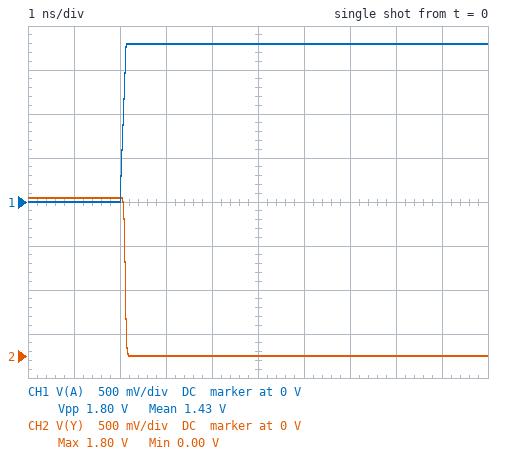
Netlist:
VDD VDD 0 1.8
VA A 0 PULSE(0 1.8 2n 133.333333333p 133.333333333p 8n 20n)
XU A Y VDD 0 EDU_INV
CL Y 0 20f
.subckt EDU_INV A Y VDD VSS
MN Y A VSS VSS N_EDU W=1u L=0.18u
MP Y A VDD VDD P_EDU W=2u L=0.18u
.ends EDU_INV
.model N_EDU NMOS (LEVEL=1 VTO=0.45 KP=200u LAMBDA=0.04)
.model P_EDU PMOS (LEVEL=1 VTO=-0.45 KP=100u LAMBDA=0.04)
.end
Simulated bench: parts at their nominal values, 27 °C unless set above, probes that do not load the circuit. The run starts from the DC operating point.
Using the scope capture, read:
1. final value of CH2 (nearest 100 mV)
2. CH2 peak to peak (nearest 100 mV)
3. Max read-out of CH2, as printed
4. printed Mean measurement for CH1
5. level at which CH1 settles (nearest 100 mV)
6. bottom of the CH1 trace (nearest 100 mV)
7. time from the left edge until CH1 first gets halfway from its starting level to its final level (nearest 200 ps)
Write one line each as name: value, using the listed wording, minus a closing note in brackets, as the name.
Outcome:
final value of CH2: 0 V
CH2 peak to peak: 1.8 V
Max read-out of CH2, as printed: 1.80 V
printed Mean measurement for CH1: 1.43 V
level at which CH1 settles: 1.8 V
bottom of the CH1 trace: 0 V
time from the left edge until CH1 first gets halfway from its starting level to its final level: 2.0 ns
